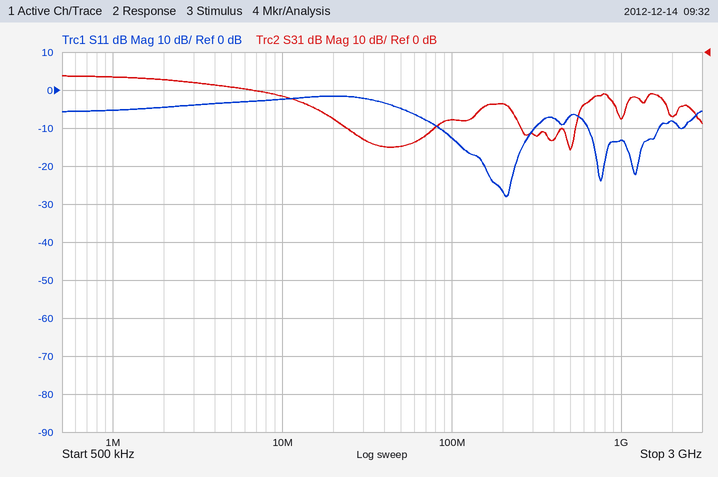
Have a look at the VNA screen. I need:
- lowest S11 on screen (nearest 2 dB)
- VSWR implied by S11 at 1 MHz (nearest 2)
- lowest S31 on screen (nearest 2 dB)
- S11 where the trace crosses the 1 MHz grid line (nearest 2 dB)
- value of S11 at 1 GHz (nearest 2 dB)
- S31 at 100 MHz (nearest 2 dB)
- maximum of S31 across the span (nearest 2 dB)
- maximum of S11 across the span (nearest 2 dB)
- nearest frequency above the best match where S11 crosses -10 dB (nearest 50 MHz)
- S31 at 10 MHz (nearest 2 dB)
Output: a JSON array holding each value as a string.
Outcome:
["-28 dB", "4", "-26 dB", "-6 dB", "-14 dB", "-18 dB", "-6 dB", "-2 dB", "300 MHz", "-12 dB"]
